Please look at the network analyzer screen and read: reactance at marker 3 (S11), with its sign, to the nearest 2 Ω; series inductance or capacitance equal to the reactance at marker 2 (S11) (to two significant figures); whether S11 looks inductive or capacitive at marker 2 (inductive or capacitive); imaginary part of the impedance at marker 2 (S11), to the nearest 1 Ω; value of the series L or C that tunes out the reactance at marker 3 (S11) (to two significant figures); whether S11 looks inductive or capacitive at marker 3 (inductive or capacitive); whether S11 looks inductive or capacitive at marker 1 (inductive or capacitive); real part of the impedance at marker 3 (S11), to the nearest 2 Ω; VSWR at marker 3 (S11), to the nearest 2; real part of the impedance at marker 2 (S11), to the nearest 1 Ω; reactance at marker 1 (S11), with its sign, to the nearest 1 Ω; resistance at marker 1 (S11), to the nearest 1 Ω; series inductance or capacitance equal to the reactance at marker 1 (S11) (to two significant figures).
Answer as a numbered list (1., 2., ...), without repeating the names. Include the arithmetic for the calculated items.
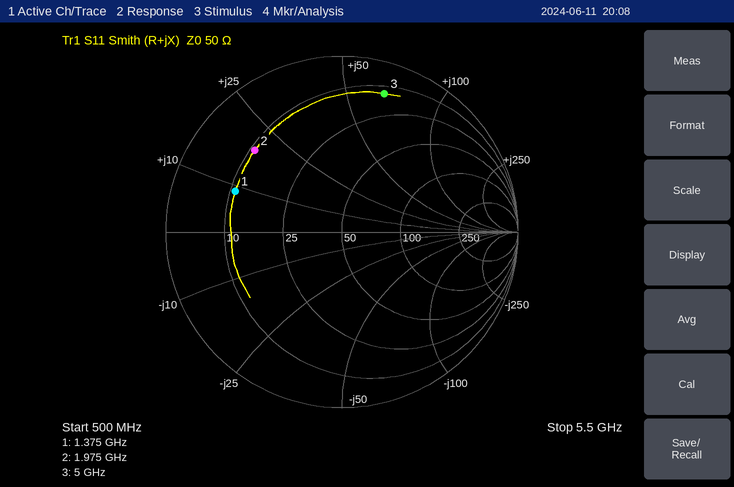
1. +66 Ω
2. L = 19 Ω/(2π × 1.975 GHz) ≈ 1.5 nH
3. inductive
4. +19 Ω
5. C = 1/(2π × 5 GHz × 66 Ω) ≈ 482 fF, so 480 fF to two significant figures
6. inductive
7. inductive
8. 14 Ω
9. 10
10. 11 Ω
11. +9 Ω
12. 11 Ω
13. L = 9 Ω/(2π × 1.375 GHz) ≈ 1.0 nH
